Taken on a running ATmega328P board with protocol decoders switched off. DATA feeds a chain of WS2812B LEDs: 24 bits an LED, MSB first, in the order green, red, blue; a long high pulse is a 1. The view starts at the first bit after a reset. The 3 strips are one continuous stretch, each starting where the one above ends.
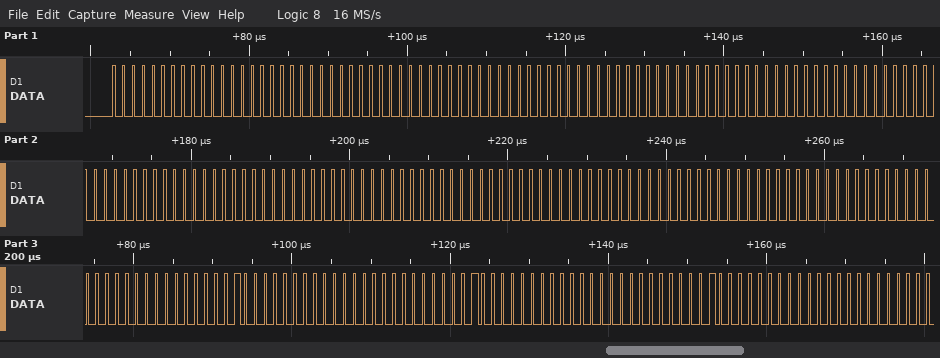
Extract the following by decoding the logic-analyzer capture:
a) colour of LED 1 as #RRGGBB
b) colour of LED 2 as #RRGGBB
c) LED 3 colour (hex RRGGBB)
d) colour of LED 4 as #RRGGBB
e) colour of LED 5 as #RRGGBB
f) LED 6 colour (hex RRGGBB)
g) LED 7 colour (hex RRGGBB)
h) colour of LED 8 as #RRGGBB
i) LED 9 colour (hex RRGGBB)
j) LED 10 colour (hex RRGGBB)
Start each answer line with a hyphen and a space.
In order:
- #000000
- #000000
- #000000
- #000000
- #000000
- #000000
- #000000
- #000080
- #000080
- #000080
